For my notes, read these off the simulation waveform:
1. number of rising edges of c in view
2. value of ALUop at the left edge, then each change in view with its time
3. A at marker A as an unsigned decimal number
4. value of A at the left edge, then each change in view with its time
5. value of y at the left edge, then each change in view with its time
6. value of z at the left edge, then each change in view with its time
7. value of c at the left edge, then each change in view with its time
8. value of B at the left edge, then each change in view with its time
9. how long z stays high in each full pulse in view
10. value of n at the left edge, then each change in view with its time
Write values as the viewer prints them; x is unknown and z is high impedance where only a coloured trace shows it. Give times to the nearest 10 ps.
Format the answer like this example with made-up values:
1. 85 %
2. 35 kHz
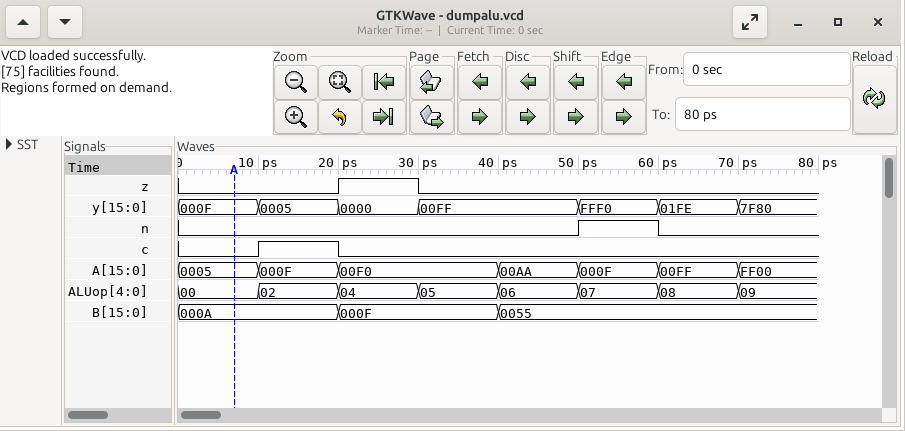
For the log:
1. 1
2. 00, 02 at 10 ps, 04 at 20 ps, 05 at 30 ps, 06 at 40 ps, 07 at 50 ps, 08 at 60 ps, 09 at 70 ps
3. 5
4. 0005, 000F at 10 ps, 00F0 at 20 ps, 00AA at 40 ps, 000F at 50 ps, 00FF at 60 ps, FF00 at 70 ps
5. 000F, 0005 at 10 ps, 0000 at 20 ps, 00FF at 30 ps, FFF0 at 50 ps, 01FE at 60 ps, 7F80 at 70 ps
6. 0, 1 at 20 ps, 0 at 30 ps
7. 0, 1 at 10 ps, 0 at 20 ps
8. 000A, 000F at 20 ps, 0055 at 40 ps
9. 10 ps
10. 0, 1 at 50 ps, 0 at 60 ps
